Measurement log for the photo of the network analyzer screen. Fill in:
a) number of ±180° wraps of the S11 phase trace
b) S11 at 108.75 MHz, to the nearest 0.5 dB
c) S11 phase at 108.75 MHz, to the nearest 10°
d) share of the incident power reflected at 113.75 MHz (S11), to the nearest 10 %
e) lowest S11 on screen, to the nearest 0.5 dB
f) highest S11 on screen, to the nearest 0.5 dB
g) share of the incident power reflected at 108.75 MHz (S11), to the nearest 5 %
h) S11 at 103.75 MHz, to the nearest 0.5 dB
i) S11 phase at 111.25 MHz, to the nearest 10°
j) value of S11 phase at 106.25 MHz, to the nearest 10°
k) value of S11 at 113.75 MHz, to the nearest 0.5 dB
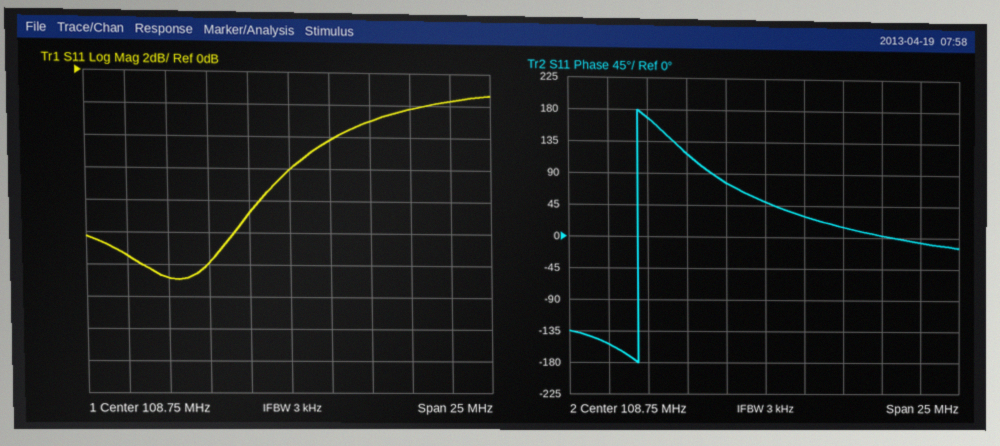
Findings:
1
-6.0 dB
50°
50 %
-13.0 dB
-1.5 dB
25 %
-12.0 dB
30°
80°
-3.0 dB
